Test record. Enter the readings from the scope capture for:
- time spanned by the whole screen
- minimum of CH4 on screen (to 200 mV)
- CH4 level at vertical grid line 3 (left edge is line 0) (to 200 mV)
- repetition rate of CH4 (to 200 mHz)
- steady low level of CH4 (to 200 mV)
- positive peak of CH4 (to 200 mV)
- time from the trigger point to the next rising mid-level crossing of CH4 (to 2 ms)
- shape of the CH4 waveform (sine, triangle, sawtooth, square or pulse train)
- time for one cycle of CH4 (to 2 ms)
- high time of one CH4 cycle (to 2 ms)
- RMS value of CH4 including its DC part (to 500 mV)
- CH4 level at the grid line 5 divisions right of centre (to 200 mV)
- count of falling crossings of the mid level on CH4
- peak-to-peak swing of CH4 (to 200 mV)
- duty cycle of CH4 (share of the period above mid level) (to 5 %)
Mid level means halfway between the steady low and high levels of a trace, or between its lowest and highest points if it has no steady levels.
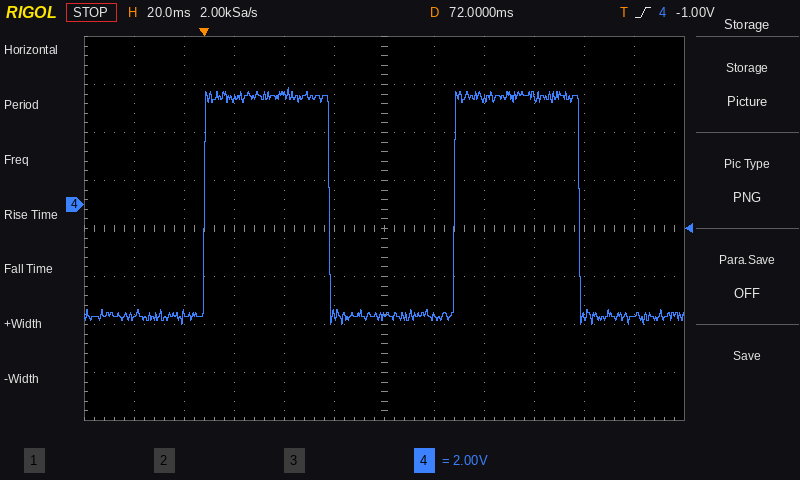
240 ms
-5.0 V
4.4 V
10.0 Hz
-4.6 V
4.8 V
100 ms
square
100 ms
50 ms
4.5 V
-4.6 V
2
9.8 V
50 %
